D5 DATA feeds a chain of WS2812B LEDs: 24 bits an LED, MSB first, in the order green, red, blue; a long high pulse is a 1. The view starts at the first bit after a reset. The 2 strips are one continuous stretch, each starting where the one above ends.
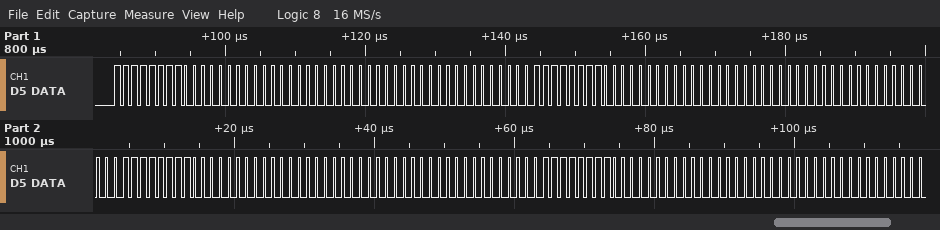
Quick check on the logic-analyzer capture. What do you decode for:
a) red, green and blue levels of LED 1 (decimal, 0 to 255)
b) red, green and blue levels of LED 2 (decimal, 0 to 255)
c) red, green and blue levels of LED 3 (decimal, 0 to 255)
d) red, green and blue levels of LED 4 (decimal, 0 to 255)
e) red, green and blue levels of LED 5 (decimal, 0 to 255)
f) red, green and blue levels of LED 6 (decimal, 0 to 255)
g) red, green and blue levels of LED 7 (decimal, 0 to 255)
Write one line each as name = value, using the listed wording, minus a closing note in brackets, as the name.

red, green and blue levels of LED 1 = 0, 255, 0
red, green and blue levels of LED 2 = 0, 0, 0
red, green and blue levels of LED 3 = 0, 255, 0
red, green and blue levels of LED 4 = 0, 0, 0
red, green and blue levels of LED 5 = 0, 255, 0
red, green and blue levels of LED 6 = 0, 0, 0
red, green and blue levels of LED 7 = 0, 255, 0
